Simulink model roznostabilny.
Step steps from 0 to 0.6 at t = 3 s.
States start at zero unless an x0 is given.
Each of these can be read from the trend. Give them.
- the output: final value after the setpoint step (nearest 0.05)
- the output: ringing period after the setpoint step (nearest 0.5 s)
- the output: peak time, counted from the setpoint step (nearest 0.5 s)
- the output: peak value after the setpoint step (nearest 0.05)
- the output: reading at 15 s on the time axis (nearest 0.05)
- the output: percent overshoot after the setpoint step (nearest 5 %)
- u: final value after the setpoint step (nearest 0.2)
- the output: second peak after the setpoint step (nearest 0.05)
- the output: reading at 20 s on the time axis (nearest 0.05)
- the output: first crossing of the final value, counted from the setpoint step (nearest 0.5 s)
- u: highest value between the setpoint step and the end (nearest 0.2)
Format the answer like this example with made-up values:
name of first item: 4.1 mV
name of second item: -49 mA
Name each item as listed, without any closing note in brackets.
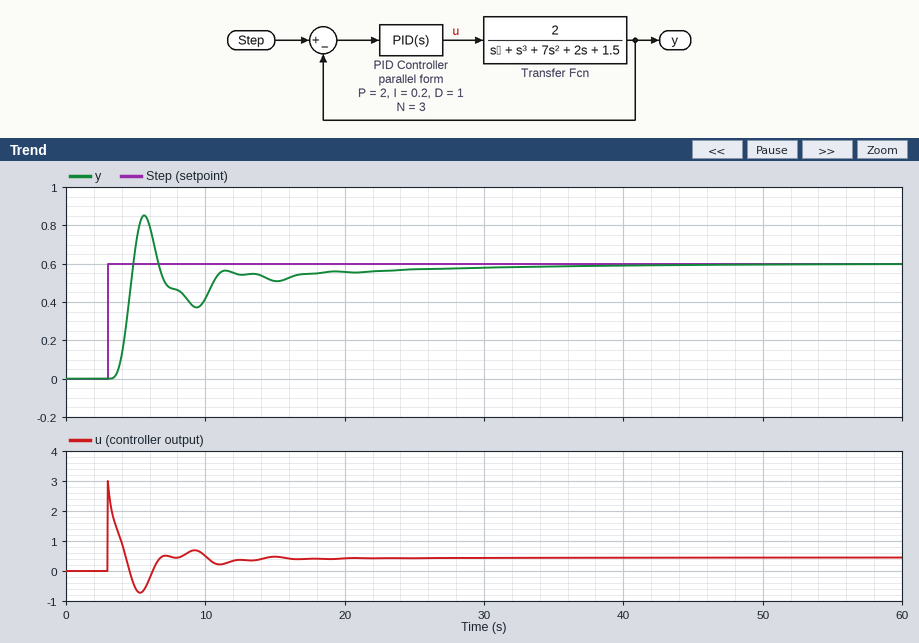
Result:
the output: final value after the setpoint step: 0.60
the output: ringing period after the setpoint step: 6.0 s
the output: peak time, counted from the setpoint step: 2.5 s
the output: peak value after the setpoint step: 0.85
the output: reading at 15 s on the time axis: 0.50
the output: percent overshoot after the setpoint step: 40 %
u: final value after the setpoint step: 0.4
the output: second peak after the setpoint step: 0.55
the output: reading at 20 s on the time axis: 0.55
the output: first crossing of the final value, counted from the setpoint step: 2.0 s
u: highest value between the setpoint step and the end: 3.0
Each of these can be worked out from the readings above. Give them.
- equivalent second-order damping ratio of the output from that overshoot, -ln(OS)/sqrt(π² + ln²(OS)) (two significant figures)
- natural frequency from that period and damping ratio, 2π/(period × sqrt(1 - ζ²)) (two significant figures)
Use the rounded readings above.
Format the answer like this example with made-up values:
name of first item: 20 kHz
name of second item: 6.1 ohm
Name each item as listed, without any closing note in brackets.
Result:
equivalent second-order damping ratio of the output from that overshoot, -ln(OS)/sqrt(π² + ln²(OS)): 0.28
natural frequency from that period and damping ratio, 2π/(period × sqrt(1 - ζ²)): 1.1 rad/s
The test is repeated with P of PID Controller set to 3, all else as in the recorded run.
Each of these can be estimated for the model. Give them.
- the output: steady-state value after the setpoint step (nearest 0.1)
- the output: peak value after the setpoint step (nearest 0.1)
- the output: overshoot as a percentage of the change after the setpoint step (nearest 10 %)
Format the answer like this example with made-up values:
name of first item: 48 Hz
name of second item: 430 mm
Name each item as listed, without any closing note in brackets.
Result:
the output: steady-state value after the setpoint step: 0.6
the output: peak value after the setpoint step: 1.1
the output: overshoot as a percentage of the change after the setpoint step: 80 %
